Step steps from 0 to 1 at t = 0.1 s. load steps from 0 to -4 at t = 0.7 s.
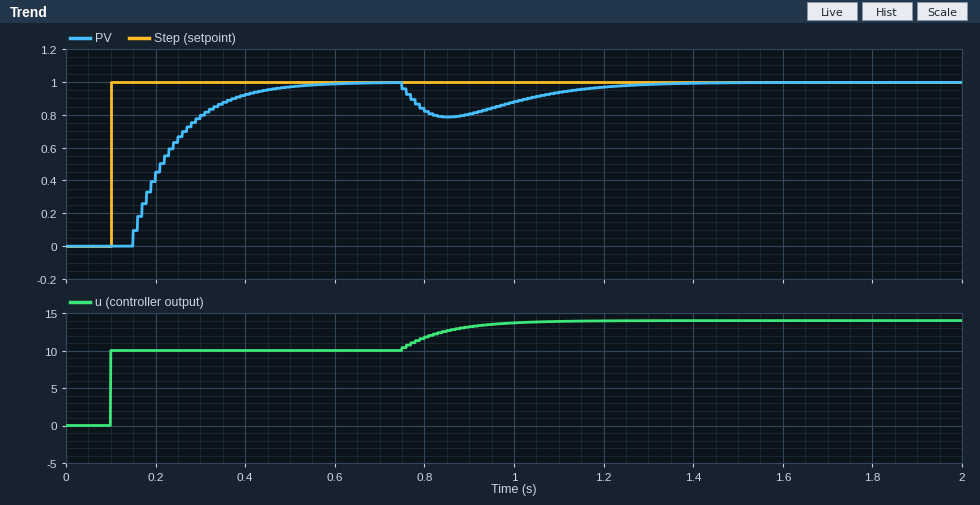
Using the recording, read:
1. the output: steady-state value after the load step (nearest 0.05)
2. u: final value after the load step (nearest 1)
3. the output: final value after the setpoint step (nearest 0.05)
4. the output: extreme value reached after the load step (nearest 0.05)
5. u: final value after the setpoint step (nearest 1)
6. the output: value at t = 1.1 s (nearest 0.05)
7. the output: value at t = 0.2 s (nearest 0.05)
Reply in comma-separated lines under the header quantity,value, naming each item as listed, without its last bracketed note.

quantity,value
the output: steady-state value after the load step,1.00
u: final value after the load step,14
the output: final value after the setpoint step,1.00
the output: extreme value reached after the load step,0.80
u: final value after the setpoint step,10
the output: value at t = 1.1 s,0.95
the output: value at t = 0.2 s,0.45
